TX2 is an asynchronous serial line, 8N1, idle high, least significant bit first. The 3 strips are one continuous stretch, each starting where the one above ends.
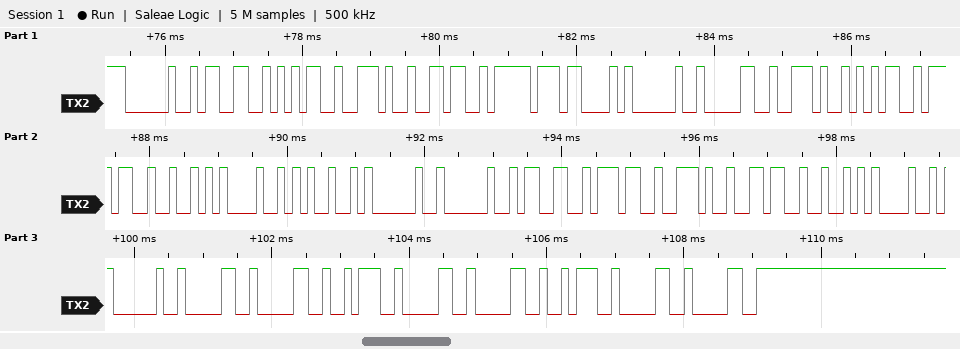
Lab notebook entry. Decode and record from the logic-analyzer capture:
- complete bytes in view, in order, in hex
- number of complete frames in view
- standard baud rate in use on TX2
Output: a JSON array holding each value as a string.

["20 33 35 2E 36 DF 43 20 30 2E 35 37 52 48 49 20 20 33 37 2E 36 52 48 20 30 30 3A 30 30 3A 30 30", "32", "9600 baud"]
